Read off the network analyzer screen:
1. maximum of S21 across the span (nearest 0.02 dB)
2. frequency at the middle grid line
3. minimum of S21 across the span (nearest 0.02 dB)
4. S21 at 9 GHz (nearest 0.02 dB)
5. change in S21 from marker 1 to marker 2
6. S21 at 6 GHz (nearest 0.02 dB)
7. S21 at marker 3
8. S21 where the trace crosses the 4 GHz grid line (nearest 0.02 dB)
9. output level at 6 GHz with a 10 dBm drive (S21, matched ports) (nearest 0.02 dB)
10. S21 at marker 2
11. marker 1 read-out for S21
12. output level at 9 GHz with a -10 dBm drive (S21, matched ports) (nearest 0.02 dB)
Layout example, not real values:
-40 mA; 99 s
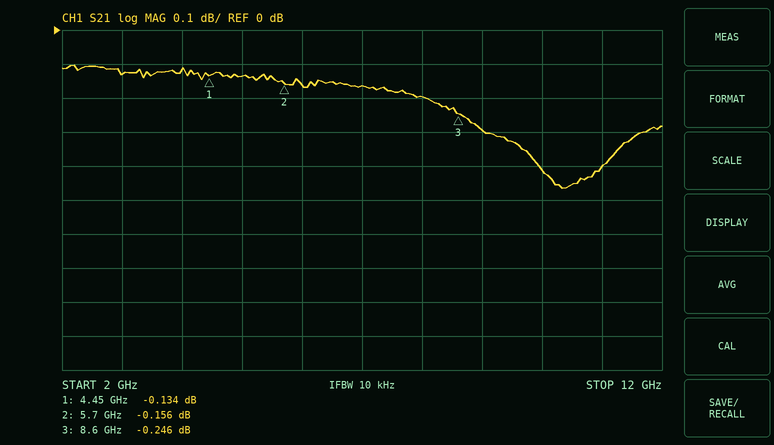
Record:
-0.10 dB; 7 GHz; -0.46 dB; -0.30 dB; -0.022 dB; -0.16 dB; -0.246 dB; -0.12 dB; 9.84 dBm; -0.156 dB; -0.134 dB; -10.30 dBm
